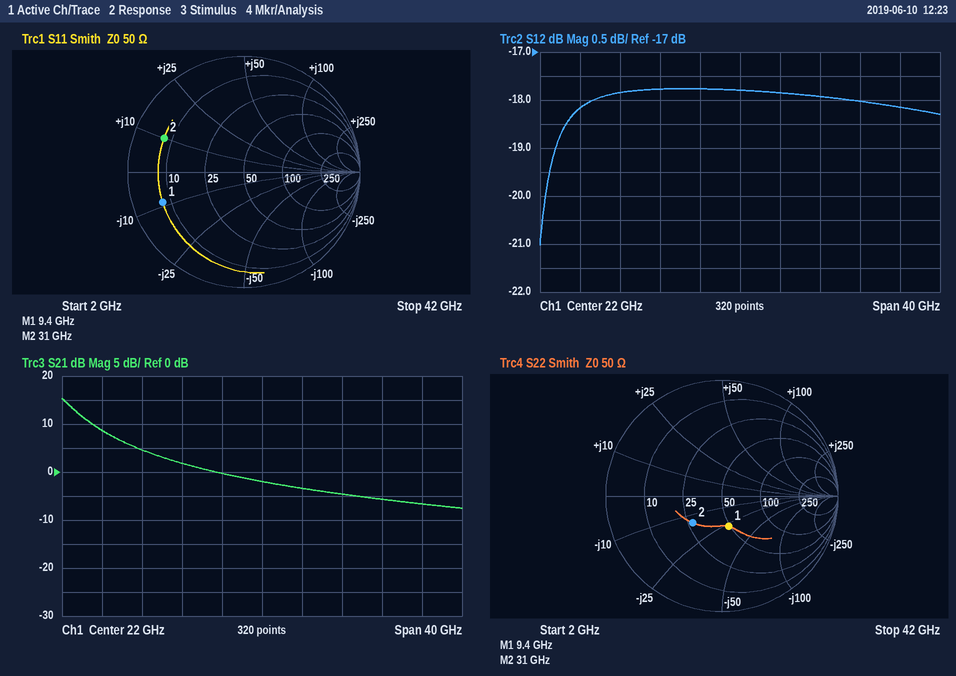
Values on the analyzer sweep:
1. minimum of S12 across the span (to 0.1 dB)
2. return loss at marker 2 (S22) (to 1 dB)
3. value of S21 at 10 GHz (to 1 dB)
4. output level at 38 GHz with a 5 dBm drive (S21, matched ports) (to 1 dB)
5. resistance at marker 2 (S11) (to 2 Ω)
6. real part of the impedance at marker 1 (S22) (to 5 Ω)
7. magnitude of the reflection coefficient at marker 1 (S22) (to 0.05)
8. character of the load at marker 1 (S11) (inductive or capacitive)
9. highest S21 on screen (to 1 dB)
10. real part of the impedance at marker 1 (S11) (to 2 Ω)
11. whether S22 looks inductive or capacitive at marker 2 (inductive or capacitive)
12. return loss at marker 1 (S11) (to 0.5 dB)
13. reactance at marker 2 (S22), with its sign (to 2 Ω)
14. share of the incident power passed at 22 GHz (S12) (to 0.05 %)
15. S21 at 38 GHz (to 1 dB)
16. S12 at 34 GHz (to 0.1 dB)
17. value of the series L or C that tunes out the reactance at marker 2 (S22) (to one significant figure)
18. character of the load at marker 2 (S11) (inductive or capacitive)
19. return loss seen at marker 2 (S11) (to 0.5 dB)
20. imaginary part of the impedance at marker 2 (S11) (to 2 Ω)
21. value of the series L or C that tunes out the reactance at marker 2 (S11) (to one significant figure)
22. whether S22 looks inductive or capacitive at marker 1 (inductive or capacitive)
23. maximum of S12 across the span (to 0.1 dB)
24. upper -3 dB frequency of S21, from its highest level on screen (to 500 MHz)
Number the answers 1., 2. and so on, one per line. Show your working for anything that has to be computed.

1. -21.0 dB
2. 9 dB
3. 5 dB
4. 5 dBm + (-7 dB) = -2 dBm
5. 8 Ω
6. 50 Ω
7. 0.25
8. capacitive
9. 15 dB
10. 8 Ω
11. capacitive
12. 2.5 dB
13. -14 Ω
14. 10^(-17.8/10) ≈ 1.66 %, so 1.65 % to the nearest 0.05 %
15. -7 dB
16. -18.0 dB
17. L = 14 Ω/(2π × 31 GHz) ≈ 71.9 pH, so 70 pH to one significant figure
18. inductive
19. 2.5 dB
20. +10 Ω
21. C = 1/(2π × 31 GHz × 10 Ω) ≈ 513 fF, so 500 fF to one significant figure
22. capacitive
23. -17.8 dB
24. 3.5 GHz
